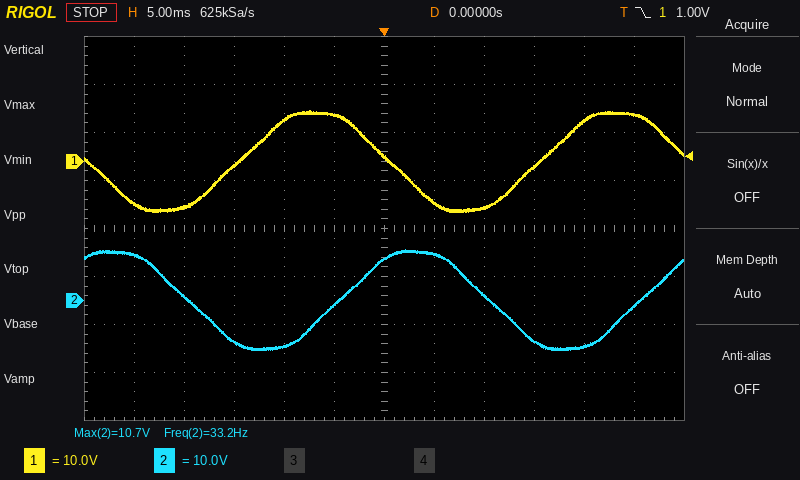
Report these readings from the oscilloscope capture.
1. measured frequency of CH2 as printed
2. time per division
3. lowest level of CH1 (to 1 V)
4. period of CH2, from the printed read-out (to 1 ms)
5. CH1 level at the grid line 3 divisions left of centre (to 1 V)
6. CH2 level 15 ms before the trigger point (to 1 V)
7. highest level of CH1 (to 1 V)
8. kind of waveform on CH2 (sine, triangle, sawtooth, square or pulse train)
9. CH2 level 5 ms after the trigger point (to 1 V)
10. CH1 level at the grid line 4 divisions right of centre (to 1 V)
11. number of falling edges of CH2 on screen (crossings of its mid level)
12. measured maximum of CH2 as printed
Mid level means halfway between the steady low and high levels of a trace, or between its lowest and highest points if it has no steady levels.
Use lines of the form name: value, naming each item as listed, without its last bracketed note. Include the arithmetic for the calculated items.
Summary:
measured frequency of CH2 as printed: 33.2 Hz
time per division: 5 ms
lowest level of CH1: -11 V
period of CH2, from the printed read-out: 1 / 33.2 Hz ≈ 30 ms
CH1 level at the grid line 3 divisions left of centre: -1 V
CH2 level 15 ms before the trigger point: -9 V
highest level of CH1: 11 V
kind of waveform on CH2: sine
CH2 level 5 ms after the trigger point: 10 V
CH1 level at the grid line 4 divisions right of centre: 8 V
number of falling edges of CH2 on screen: 2
measured maximum of CH2 as printed: 10.7 V
